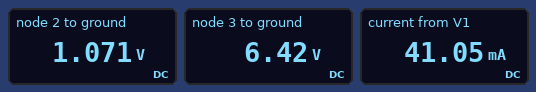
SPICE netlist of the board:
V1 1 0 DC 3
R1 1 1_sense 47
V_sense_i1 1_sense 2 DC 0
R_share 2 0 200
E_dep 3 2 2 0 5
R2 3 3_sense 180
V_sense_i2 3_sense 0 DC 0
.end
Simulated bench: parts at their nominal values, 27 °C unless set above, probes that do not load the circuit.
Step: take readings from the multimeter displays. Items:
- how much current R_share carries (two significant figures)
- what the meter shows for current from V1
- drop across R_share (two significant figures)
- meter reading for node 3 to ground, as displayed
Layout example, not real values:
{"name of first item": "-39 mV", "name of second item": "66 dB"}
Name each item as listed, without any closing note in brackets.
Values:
{"how much current R_share carries": "5.4 mA", "what the meter shows for current from V1": "41.05 mA", "drop across R_share": "1.1 V", "meter reading for node 3 to ground, as displayed": "6.42 V"}
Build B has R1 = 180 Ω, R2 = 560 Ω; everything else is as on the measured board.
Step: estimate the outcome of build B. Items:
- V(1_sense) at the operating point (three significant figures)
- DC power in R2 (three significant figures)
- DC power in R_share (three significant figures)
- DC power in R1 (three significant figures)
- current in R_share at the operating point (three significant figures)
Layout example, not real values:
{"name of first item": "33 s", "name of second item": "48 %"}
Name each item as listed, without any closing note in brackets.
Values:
{"V(1_sense) at the operating point": "784 mV", "DC power in R2": "39.5 mW", "DC power in R_share": "3.07 mW", "DC power in R1": "27.3 mW", "current in R_share at the operating point": "3.92 mA"}
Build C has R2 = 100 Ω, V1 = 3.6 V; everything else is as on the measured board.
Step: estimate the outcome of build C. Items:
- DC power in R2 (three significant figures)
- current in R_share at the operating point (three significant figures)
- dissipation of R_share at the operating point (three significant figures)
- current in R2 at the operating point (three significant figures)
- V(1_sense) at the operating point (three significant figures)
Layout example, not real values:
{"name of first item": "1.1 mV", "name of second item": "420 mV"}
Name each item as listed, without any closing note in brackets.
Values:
{"DC power in R2": "284 mW", "current in R_share at the operating point": "4.44 mA", "dissipation of R_share at the operating point": "3.94 mW", "current in R2 at the operating point": "53.3 mA", "V(1_sense) at the operating point": "888 mV"}
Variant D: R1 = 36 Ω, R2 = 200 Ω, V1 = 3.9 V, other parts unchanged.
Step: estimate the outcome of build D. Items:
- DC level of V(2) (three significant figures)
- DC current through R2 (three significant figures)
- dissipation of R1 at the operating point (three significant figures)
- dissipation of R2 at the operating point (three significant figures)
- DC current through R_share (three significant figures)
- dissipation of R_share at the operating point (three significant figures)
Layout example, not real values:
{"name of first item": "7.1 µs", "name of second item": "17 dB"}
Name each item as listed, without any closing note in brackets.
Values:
{"DC level of V(2)": "1.73 V", "DC current through R2": "51.8 mA", "dissipation of R1 at the operating point": "131 mW", "dissipation of R2 at the operating point": "536 mW", "DC current through R_share": "8.63 mA", "dissipation of R_share at the operating point": "14.9 mW"}
